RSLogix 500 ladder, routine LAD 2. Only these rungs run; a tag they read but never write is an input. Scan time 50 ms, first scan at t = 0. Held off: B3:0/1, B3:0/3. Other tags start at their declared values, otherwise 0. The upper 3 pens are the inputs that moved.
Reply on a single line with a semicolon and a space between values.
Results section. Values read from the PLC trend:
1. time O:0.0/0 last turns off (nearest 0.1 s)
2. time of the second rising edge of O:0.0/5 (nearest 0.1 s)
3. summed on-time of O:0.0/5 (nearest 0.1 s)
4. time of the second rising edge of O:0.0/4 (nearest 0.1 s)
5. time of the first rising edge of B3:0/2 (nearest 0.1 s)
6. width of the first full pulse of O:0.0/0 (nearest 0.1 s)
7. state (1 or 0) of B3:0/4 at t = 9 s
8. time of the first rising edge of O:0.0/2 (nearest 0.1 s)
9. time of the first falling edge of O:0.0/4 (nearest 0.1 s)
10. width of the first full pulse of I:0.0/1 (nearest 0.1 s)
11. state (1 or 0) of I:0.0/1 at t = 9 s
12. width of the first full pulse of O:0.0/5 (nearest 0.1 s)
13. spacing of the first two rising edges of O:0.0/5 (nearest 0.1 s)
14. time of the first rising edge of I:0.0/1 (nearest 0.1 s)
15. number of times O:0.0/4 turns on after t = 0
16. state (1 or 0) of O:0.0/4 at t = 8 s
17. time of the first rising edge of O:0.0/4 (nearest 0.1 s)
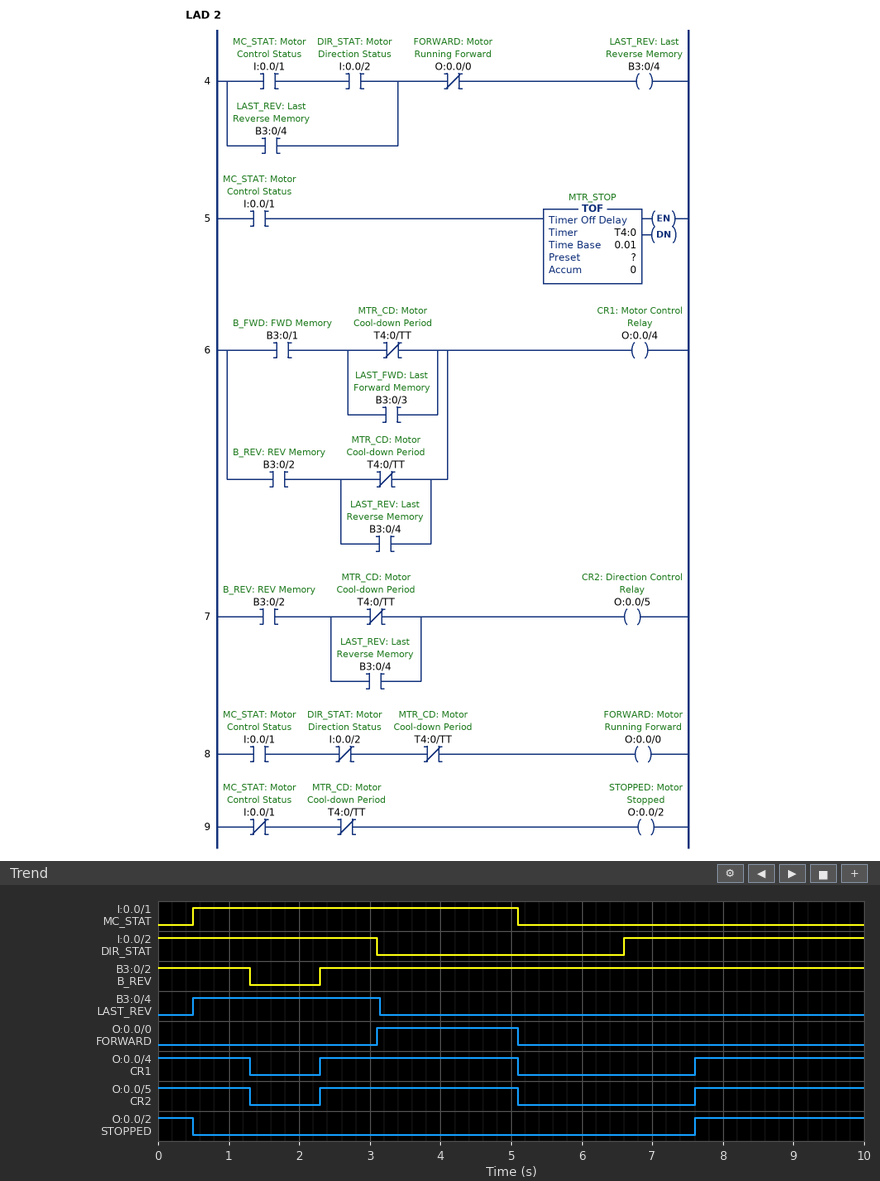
5.1 s; 7.6 s; 6.5 s; 7.6 s; 2.3 s; 2.0 s; 0; 7.6 s; 1.3 s; 4.6 s; 0; 2.8 s; 5.3 s; 0.5 s; 2; 1; 2.3 s
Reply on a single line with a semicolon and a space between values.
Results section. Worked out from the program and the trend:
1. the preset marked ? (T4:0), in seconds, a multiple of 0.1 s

2.5 s
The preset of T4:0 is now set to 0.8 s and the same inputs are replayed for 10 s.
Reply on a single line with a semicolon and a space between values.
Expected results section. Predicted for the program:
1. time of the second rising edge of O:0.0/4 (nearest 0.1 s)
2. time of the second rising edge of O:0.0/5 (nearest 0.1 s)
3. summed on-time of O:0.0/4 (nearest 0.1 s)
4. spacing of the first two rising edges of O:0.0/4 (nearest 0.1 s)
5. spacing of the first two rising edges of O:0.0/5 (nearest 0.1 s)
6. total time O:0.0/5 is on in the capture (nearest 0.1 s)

5.9 s; 5.9 s; 8.2 s; 3.6 s; 3.6 s; 8.2 s
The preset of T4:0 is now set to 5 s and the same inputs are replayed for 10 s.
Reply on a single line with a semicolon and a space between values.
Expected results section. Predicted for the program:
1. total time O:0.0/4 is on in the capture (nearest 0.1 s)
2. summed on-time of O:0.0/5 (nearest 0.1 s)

4.1 s; 4.1 s
